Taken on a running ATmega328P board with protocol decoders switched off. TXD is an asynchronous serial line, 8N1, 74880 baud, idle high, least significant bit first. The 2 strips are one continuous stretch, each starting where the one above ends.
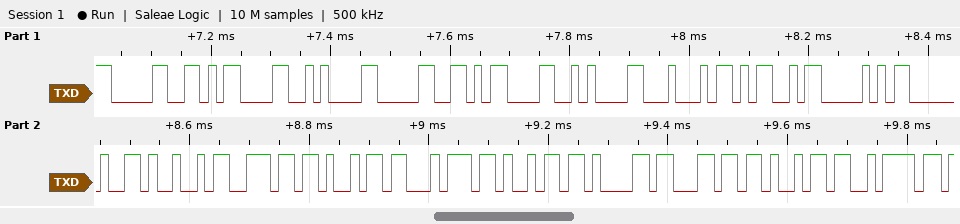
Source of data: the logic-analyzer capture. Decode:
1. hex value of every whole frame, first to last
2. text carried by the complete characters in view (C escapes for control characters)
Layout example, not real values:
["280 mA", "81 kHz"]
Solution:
["30 0D 0A 30 0D 0A 44 4D 50 20 49 6E 69 74 69 61 6C 69 7A", "\"0\\r\\n0\\r\\nDMP Initializ\""]
